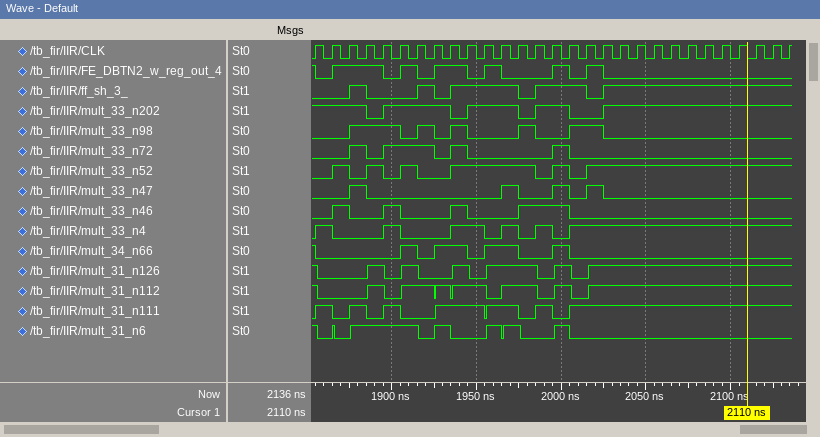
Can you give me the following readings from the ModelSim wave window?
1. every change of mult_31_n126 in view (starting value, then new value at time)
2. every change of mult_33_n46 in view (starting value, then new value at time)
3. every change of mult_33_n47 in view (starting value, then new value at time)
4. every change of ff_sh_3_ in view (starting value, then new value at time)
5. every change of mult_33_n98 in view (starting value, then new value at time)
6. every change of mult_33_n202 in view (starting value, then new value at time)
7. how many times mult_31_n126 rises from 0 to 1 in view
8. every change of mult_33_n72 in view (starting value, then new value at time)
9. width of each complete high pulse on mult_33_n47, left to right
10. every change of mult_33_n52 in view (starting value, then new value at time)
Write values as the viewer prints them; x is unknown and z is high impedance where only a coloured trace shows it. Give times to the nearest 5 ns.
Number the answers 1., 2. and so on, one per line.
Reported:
1. 1, 0 at 1855 ns, 1 at 1885 ns, 0 at 1895 ns, 1 at 1905 ns, 0 at 1915 ns, 1 at 1935 ns, 0 at 1945 ns, 1 at 1955 ns, 0 at 1985 ns, 1 at 1995 ns, 0 at 2005 ns, 1 at 2015 ns
2. 0, 1 at 1865 ns, 0 at 1875 ns, 1 at 1895 ns, 0 at 1905 ns, 1 at 1935 ns, 0 at 1945 ns, 1 at 1975 ns, 0 at 2005 ns
3. 0, 1 at 1875 ns, 0 at 1885 ns, 1 at 1965 ns, 0 at 1975 ns, 1 at 1995 ns, 0 at 2005 ns, 1 at 2015 ns, 0 at 2025 ns
4. 0, 1 at 1875 ns, 0 at 1885 ns, 1 at 1915 ns, 0 at 1925 ns, 1 at 1935 ns, 0 at 1975 ns, 1 at 1985 ns, 0 at 2015 ns, 1 at 2025 ns
5. 0, 1 at 1875 ns, 0 at 1905 ns, 1 at 1915 ns, 0 at 1925 ns, 1 at 1935 ns, 0 at 1945 ns, 1 at 1975 ns, 0 at 1985 ns, 1 at 2005 ns, 0 at 2025 ns
6. 1, 0 at 1885 ns, 1 at 1895 ns, 0 at 1935 ns, 1 at 1945 ns, 0 at 1975 ns, 1 at 1985 ns, 0 at 2005 ns, 1 at 2025 ns
7. 6
8. 0, 1 at 1875 ns, 0 at 1885 ns, 1 at 1895 ns, 0 at 1925 ns, 1 at 1935 ns, 0 at 1945 ns, 1 at 1995 ns, 0 at 2005 ns
9. 10 ns, 10 ns, 10 ns, 10 ns
10. 0, 1 at 1865 ns, 0 at 1875 ns, 1 at 1885 ns, 0 at 1895 ns, 1 at 1905 ns, 0 at 1915 ns, 1 at 1935 ns, 0 at 1985 ns, 1 at 1995 ns, 0 at 2005 ns, 1 at 2015 ns
